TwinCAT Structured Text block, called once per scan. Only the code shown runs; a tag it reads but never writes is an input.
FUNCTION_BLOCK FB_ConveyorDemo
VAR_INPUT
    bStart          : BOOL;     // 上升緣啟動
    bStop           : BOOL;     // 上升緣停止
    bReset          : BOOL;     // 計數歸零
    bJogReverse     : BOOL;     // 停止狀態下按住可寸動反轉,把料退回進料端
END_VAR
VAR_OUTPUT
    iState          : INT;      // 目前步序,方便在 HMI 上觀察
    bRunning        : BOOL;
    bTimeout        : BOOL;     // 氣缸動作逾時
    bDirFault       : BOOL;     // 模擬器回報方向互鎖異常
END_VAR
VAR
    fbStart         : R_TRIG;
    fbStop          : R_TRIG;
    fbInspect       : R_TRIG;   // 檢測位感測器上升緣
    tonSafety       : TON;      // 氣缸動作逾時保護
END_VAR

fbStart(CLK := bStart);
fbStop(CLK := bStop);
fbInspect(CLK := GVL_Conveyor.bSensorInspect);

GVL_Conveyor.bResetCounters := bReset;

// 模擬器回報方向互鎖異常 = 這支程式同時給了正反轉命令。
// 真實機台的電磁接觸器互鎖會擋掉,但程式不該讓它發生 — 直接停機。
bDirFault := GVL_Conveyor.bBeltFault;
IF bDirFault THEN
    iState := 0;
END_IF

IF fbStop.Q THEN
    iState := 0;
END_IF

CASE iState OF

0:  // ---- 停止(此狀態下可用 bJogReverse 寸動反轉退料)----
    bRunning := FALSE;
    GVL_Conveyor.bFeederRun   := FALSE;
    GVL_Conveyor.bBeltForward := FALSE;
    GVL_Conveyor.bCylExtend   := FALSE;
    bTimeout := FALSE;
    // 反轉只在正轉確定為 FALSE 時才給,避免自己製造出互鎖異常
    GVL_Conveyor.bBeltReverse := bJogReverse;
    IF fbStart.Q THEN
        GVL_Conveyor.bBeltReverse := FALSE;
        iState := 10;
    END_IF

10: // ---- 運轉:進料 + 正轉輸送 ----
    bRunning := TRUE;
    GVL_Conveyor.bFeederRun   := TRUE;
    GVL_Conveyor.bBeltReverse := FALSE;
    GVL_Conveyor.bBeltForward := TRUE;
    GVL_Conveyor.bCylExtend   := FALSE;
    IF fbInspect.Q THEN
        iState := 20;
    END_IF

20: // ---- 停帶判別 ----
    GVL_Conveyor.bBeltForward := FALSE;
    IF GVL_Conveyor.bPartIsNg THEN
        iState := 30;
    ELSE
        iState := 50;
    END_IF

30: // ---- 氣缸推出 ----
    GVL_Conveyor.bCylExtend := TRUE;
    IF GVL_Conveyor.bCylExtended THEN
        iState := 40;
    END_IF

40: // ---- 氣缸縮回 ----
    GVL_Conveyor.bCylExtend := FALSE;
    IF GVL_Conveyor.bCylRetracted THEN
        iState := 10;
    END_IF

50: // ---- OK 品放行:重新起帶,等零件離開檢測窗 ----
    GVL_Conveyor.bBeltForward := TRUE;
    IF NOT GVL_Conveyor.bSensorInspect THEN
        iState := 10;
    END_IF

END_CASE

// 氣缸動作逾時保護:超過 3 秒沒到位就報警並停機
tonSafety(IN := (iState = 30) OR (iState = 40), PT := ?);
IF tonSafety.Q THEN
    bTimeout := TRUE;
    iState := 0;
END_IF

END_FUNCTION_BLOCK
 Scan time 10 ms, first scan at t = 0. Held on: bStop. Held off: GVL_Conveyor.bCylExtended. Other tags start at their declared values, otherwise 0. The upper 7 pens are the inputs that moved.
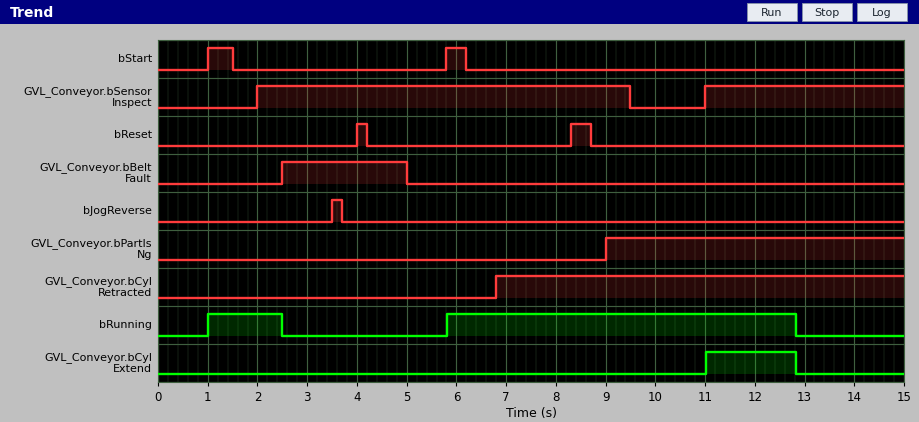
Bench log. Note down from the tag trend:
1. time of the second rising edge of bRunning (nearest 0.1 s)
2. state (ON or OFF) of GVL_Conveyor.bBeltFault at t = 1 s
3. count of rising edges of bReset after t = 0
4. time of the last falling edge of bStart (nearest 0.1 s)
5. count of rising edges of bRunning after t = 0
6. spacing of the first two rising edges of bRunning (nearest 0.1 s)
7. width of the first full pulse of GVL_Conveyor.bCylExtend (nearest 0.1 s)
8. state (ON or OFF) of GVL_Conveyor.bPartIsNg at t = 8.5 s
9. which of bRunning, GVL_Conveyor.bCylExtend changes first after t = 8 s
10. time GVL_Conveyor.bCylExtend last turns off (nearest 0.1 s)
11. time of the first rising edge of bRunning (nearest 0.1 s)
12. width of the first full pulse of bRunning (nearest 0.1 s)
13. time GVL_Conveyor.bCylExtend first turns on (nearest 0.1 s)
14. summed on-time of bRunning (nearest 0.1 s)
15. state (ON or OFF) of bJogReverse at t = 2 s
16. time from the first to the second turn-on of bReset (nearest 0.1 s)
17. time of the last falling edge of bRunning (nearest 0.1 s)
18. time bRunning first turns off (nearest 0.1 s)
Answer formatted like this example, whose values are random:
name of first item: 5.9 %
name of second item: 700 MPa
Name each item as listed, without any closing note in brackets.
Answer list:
time of the second rising edge of bRunning: 5.8 s
state (ON or OFF) of GVL_Conveyor.bBeltFault at t = 1 s: OFF
count of rising edges of bReset after t = 0: 2
time of the last falling edge of bStart: 6.2 s
count of rising edges of bRunning after t = 0: 2
spacing of the first two rising edges of bRunning: 4.8 s
width of the first full pulse of GVL_Conveyor.bCylExtend: 1.8 s
state (ON or OFF) of GVL_Conveyor.bPartIsNg at t = 8.5 s: OFF
which of bRunning, GVL_Conveyor.bCylExtend changes first after t = 8 s: GVL_Conveyor.bCylExtend
time GVL_Conveyor.bCylExtend last turns off: 12.8 s
time of the first rising edge of bRunning: 1.0 s
width of the first full pulse of bRunning: 1.5 s
time GVL_Conveyor.bCylExtend first turns on: 11.0 s
summed on-time of bRunning: 8.5 s
state (ON or OFF) of bJogReverse at t = 2 s: OFF
time from the first to the second turn-on of bReset: 4.3 s
time of the last falling edge of bRunning: 12.8 s
time bRunning first turns off: 2.5 s
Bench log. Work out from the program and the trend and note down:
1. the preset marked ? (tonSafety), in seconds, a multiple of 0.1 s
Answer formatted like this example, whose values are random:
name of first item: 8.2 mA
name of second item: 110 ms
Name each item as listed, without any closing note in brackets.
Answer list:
the preset marked ? (tonSafety), in seconds, a multiple of 0.1 s: 1.8 s
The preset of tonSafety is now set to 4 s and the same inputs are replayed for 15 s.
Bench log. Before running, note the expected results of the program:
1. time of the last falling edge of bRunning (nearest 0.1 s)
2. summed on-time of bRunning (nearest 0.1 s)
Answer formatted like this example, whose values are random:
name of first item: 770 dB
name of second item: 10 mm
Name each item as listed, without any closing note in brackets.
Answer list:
time of the last falling edge of bRunning: 2.5 s
summed on-time of bRunning: 10.7 s
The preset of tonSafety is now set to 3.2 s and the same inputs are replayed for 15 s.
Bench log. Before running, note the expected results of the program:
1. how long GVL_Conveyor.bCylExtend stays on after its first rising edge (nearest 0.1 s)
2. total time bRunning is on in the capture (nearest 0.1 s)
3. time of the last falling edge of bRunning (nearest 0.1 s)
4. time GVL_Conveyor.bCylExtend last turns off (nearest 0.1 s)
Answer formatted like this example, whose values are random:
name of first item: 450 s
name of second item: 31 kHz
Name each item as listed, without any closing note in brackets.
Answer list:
how long GVL_Conveyor.bCylExtend stays on after its first rising edge: 3.2 s
total time bRunning is on in the capture: 9.9 s
time of the last falling edge of bRunning: 14.2 s
time GVL_Conveyor.bCylExtend last turns off: 14.2 s
